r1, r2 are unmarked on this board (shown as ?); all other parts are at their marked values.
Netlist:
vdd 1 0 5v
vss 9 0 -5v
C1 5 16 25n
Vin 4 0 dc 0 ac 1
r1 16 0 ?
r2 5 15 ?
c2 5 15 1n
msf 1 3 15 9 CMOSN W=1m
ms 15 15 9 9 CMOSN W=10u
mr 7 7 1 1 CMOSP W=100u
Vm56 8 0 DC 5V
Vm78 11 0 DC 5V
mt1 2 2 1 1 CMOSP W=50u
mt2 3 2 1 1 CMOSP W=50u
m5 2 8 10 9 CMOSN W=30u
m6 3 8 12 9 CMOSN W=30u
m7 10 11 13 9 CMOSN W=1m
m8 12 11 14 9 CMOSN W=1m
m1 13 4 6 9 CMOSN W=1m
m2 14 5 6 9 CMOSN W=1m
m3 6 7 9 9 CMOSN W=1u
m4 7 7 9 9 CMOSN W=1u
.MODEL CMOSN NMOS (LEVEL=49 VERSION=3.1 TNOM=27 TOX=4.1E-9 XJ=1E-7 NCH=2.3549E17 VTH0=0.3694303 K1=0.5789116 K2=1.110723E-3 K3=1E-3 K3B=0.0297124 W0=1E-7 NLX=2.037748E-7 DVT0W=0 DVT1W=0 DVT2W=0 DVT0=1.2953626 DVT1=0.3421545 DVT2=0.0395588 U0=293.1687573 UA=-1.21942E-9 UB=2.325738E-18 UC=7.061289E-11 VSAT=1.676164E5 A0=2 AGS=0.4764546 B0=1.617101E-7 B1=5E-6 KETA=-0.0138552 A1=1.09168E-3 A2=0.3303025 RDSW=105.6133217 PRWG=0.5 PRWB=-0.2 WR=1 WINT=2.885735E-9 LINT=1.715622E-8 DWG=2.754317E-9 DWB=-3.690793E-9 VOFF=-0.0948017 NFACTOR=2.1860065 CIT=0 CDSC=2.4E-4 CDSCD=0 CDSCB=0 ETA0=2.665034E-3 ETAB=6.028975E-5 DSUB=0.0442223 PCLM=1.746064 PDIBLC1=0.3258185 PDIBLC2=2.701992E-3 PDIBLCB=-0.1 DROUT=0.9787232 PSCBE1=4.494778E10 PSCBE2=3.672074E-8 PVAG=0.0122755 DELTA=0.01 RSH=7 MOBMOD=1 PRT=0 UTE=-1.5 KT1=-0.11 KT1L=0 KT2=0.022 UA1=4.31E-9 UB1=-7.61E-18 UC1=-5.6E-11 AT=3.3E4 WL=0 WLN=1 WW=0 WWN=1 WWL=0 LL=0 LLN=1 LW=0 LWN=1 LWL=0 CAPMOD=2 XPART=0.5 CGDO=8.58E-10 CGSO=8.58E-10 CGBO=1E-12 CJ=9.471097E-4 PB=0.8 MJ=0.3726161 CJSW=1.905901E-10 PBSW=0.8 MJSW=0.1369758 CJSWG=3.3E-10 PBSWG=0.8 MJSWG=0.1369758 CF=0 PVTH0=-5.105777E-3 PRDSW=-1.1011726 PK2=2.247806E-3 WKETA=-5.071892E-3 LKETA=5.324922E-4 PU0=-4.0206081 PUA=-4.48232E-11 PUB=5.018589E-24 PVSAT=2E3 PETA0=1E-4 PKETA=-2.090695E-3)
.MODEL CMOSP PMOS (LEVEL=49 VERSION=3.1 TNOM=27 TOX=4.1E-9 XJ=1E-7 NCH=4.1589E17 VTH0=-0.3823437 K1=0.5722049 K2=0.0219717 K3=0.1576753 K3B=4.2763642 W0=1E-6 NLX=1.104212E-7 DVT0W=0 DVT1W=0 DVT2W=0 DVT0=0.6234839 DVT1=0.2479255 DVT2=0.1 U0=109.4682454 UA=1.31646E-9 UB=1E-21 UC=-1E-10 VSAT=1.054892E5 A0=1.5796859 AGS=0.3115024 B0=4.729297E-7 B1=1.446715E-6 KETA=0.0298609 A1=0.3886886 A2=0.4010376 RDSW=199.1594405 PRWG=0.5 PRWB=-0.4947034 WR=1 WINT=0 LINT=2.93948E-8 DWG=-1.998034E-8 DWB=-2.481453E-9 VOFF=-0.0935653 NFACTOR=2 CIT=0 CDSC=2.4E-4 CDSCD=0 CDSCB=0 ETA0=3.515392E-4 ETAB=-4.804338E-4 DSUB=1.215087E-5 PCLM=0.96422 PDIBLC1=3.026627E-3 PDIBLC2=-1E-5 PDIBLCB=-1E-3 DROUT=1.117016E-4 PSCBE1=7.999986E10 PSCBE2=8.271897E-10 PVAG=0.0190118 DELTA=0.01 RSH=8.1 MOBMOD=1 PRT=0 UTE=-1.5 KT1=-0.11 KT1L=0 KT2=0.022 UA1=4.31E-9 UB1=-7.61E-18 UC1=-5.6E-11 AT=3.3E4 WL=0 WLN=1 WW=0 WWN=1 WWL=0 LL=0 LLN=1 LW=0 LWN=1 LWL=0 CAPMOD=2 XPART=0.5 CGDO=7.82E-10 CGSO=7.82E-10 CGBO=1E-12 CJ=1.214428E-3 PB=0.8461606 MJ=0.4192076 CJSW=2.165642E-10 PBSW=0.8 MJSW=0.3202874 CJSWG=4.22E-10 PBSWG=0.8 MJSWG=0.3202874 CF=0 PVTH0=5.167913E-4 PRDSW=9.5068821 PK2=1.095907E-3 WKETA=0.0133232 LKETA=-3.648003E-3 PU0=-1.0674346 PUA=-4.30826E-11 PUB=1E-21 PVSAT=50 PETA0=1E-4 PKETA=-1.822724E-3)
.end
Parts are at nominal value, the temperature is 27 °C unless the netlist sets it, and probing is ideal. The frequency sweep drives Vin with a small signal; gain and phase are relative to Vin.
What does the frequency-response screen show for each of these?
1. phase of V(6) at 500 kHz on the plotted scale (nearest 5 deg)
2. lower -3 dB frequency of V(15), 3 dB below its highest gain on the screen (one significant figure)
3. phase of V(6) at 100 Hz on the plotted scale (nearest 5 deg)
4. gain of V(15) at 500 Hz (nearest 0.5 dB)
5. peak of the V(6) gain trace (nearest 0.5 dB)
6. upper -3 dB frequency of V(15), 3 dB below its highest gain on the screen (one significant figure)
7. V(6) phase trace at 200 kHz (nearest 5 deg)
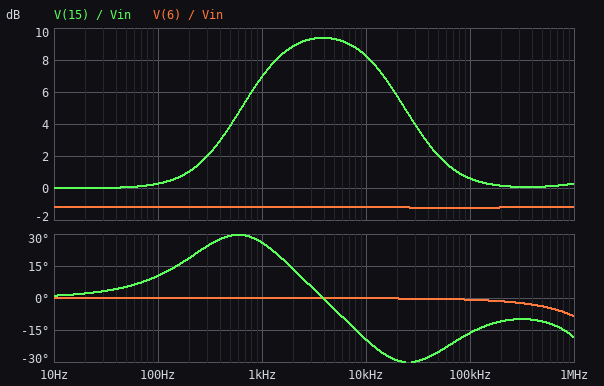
-5 deg
900 Hz
0 deg
4.0 dB
-1.0 dB
20 kHz
0 deg
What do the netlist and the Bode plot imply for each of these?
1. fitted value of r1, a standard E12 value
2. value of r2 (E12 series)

5.6 kΩ
12 kΩ
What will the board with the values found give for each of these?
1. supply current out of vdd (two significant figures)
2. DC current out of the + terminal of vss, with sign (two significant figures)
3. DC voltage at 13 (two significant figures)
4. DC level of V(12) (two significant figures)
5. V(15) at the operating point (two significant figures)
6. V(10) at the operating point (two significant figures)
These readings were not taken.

3.0 mA
-3.0 mA
3.1 V
1.5 V
4.7 mV
3.1 V
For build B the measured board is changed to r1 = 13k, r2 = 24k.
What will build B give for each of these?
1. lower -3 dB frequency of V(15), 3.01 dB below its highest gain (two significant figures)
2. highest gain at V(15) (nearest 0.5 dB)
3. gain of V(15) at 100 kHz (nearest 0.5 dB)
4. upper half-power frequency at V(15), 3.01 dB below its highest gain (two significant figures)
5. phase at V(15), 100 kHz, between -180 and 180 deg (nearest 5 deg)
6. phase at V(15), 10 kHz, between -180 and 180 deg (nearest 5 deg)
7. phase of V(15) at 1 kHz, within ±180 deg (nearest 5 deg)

370 Hz
8.5 dB
0 dB
8.7 kHz
-10 deg
-25 deg
10 deg
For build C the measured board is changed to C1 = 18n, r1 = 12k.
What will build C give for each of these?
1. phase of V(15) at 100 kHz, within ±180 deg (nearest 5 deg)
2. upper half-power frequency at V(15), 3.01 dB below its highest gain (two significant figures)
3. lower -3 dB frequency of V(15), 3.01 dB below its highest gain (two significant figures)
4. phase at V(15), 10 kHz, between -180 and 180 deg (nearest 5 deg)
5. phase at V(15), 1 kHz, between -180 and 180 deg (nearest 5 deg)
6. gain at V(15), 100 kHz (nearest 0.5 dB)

-10 deg
21 kHz
470 Hz
-15 deg
15 deg
0 dB
